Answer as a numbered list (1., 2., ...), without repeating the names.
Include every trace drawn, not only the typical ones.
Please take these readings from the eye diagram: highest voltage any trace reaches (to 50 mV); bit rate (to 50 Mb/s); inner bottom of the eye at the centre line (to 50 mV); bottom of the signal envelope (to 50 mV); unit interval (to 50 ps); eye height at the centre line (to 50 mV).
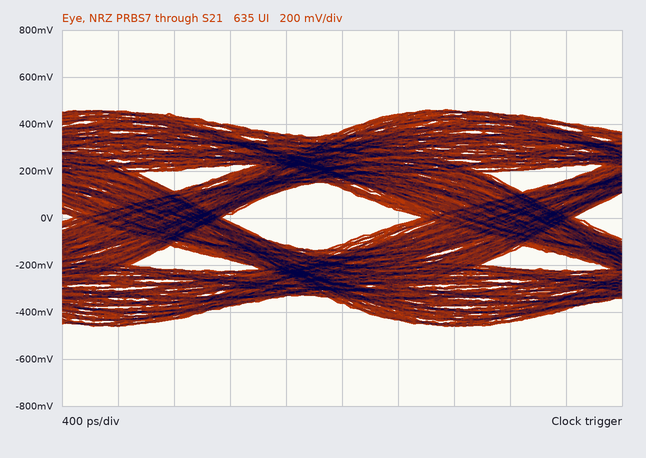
1. 450 mV
2. 400 Mb/s
3. -100 mV
4. -450 mV
5. 2.50 ns
6. 250 mV
